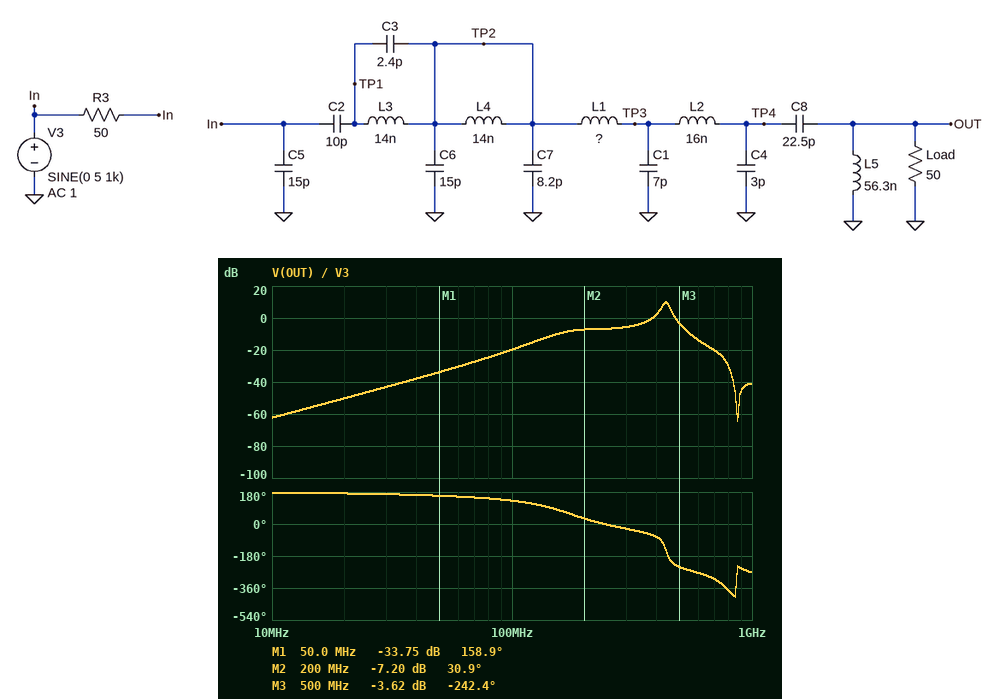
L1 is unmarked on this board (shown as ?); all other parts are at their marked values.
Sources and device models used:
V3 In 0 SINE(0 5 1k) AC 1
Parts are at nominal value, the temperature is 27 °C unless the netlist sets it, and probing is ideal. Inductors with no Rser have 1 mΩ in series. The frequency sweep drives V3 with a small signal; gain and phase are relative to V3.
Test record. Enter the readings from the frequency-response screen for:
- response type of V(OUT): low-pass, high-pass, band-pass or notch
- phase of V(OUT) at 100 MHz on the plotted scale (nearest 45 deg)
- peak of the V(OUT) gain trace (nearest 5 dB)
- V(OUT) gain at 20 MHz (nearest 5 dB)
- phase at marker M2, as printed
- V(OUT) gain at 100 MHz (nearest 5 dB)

band-pass
135 deg
10 dB
-50 dB
30.9 deg
-20 dB
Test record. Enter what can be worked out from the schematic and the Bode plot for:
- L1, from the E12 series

12 nH
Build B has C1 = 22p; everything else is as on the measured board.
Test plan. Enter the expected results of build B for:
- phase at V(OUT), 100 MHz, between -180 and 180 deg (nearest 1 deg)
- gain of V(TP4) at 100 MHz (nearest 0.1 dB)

130 deg
-16.3 dB
